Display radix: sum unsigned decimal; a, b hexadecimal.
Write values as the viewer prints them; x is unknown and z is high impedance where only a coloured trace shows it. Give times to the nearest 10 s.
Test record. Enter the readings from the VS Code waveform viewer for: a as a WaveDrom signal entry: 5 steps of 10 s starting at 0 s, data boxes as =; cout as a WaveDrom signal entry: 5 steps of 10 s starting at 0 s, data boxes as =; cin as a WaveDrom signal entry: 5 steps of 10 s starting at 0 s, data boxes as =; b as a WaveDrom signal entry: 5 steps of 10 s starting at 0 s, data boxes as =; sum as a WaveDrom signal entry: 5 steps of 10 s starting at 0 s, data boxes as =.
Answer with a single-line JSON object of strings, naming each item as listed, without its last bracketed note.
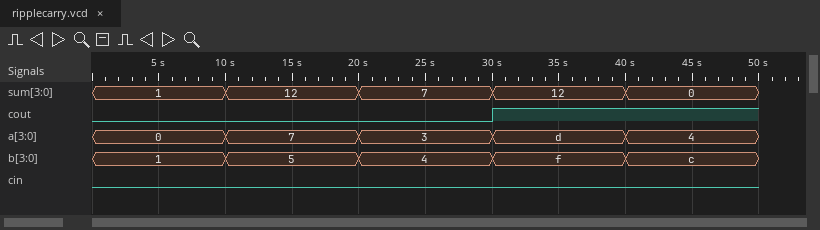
{"a as a WaveDrom signal entry: 5 steps of 10 s starting at 0 s, data boxes as =": "{name: 'a', wave: '=====', data: '0 7 3 d 4'}", "cout as a WaveDrom signal entry: 5 steps of 10 s starting at 0 s, data boxes as =": "{name: 'cout', wave: '0..1.'}", "cin as a WaveDrom signal entry: 5 steps of 10 s starting at 0 s, data boxes as =": "{name: 'cin', wave: '0....'}", "b as a WaveDrom signal entry: 5 steps of 10 s starting at 0 s, data boxes as =": "{name: 'b', wave: '=====', data: '1 5 4 f c'}", "sum as a WaveDrom signal entry: 5 steps of 10 s starting at 0 s, data boxes as =": "{name: 'sum', wave: '=====', data: '1 12 7 12 0'}"}
